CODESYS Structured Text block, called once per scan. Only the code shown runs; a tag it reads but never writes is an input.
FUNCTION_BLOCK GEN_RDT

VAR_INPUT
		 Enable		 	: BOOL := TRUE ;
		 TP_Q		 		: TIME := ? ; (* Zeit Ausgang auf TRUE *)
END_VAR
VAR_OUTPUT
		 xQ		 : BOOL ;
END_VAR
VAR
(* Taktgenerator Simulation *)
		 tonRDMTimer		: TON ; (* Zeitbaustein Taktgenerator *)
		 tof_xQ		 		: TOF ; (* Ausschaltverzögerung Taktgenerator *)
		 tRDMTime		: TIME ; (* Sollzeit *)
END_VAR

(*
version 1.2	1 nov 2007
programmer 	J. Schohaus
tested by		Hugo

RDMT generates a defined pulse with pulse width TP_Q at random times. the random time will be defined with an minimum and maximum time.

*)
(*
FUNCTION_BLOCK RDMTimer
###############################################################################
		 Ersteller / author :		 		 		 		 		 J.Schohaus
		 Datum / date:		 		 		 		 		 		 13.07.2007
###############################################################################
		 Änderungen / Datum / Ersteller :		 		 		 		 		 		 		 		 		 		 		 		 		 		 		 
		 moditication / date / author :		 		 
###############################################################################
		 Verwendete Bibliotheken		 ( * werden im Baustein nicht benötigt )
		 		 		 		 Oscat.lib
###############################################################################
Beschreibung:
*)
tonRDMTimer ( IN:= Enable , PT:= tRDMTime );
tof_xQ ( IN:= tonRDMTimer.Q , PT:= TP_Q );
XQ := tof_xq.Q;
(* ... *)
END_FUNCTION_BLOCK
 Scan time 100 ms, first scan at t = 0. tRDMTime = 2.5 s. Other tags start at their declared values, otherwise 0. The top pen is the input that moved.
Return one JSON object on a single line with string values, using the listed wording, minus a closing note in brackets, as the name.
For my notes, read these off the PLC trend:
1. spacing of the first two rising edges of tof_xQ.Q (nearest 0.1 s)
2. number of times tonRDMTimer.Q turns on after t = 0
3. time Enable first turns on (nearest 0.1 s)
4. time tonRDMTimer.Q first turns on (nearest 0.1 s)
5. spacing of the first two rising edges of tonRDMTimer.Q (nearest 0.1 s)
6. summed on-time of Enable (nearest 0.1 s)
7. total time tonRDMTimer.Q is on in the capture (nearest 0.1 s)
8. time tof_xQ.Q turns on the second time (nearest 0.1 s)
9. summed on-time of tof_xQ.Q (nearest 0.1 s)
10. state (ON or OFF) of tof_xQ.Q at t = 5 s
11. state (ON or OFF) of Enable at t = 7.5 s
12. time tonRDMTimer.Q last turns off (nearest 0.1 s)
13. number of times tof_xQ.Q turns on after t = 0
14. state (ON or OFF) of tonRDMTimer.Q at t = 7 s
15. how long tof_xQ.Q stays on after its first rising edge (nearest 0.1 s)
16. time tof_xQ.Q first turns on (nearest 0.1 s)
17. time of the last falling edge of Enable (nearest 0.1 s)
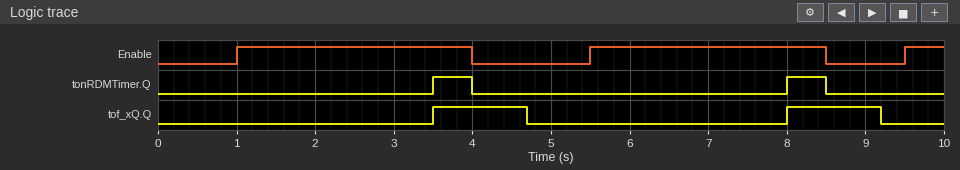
{"spacing of the first two rising edges of tof_xQ.Q": "4.5 s", "number of times tonRDMTimer.Q turns on after t = 0": "2", "time Enable first turns on": "1.0 s", "time tonRDMTimer.Q first turns on": "3.5 s", "spacing of the first two rising edges of tonRDMTimer.Q": "4.5 s", "summed on-time of Enable": "6.5 s", "total time tonRDMTimer.Q is on in the capture": "1.0 s", "time tof_xQ.Q turns on the second time": "8.0 s", "summed on-time of tof_xQ.Q": "2.4 s", "state (ON or OFF) of tof_xQ.Q at t = 5 s": "OFF", "state (ON or OFF) of Enable at t = 7.5 s": "ON", "time tonRDMTimer.Q last turns off": "8.5 s", "number of times tof_xQ.Q turns on after t = 0": "2", "state (ON or OFF) of tonRDMTimer.Q at t = 7 s": "OFF", "how long tof_xQ.Q stays on after its first rising edge": "1.2 s", "time tof_xQ.Q first turns on": "3.5 s", "time of the last falling edge of Enable": "8.5 s"}
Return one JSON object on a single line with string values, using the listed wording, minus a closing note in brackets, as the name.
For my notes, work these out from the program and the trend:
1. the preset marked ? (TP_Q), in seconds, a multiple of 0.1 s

{"the preset marked ? (TP_Q), in seconds, a multiple of 0.1 s": "0.7 s"}
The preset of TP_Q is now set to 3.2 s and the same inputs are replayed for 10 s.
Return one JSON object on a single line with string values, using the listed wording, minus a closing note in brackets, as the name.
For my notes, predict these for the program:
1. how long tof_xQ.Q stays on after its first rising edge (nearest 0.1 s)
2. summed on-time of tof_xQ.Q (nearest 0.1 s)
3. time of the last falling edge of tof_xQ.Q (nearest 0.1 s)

{"how long tof_xQ.Q stays on after its first rising edge": "3.7 s", "summed on-time of tof_xQ.Q": "5.7 s", "time of the last falling edge of tof_xQ.Q": "7.2 s"}
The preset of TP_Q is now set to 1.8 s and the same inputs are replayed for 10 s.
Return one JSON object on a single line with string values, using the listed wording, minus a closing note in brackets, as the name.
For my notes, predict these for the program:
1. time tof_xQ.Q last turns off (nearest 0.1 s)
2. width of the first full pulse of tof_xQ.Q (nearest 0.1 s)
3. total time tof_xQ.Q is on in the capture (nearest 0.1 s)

{"time tof_xQ.Q last turns off": "5.8 s", "width of the first full pulse of tof_xQ.Q": "2.3 s", "total time tof_xQ.Q is on in the capture": "4.3 s"}
